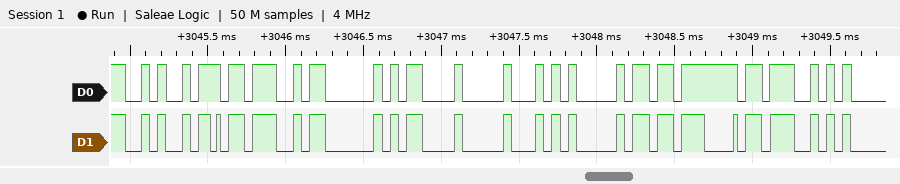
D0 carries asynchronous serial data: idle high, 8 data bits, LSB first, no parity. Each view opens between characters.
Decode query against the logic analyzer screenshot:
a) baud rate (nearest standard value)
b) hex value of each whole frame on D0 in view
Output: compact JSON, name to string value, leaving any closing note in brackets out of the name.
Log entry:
{"baud rate": "19200 baud", "hex value of each whole frame on D0 in view": "4A, 3B, 03, 0D, 10, 05, DB, 3B"}
